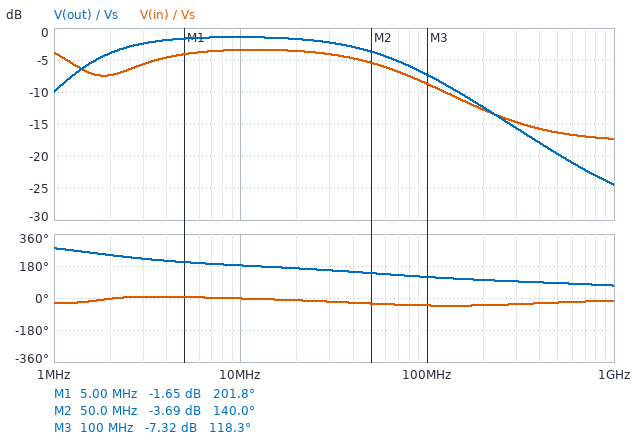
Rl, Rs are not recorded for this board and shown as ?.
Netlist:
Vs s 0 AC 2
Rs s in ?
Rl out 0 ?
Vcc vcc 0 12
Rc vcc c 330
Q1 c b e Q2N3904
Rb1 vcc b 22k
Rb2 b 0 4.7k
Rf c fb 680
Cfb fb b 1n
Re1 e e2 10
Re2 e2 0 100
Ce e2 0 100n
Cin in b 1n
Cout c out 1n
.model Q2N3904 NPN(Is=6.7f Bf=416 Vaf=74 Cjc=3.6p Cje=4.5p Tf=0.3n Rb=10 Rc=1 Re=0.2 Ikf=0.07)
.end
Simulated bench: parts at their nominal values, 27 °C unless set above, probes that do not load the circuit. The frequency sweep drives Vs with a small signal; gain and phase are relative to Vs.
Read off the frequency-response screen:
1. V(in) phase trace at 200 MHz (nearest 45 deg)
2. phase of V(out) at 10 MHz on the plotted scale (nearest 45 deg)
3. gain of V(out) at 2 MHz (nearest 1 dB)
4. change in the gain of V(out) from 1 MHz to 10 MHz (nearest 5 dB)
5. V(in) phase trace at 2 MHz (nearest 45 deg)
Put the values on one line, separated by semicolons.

-45 deg; 180 deg; -4 dB; 10 dB; 0 deg
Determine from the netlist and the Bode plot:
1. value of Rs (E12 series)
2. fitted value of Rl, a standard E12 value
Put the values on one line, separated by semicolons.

120 Ω; 18 Ω
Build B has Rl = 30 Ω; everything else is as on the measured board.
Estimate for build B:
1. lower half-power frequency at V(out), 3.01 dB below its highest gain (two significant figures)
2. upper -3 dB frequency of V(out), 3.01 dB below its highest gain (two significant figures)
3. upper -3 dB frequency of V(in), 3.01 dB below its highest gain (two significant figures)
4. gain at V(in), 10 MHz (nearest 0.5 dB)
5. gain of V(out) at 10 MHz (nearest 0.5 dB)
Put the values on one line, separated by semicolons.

1.7 MHz; 62 MHz; 880 kHz; -4.0 dB; 2.0 dB
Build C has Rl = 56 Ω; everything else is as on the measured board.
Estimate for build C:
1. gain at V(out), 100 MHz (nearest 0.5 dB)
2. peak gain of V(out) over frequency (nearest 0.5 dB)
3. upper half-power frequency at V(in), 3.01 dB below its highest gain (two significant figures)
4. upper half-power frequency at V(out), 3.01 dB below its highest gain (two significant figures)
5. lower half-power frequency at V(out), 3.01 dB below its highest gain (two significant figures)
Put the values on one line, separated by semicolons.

0 dB; 5.0 dB; 890 kHz; 67 MHz; 1.5 MHz
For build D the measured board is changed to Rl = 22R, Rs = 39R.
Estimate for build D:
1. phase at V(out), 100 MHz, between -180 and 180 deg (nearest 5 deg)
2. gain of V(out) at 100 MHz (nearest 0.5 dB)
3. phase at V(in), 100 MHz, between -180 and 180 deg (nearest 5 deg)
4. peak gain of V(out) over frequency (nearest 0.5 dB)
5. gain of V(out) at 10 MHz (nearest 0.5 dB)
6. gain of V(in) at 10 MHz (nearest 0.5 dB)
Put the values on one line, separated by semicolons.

135 deg; -0.5 dB; -25 deg; 2.5 dB; 2.0 dB; -1.5 dB
